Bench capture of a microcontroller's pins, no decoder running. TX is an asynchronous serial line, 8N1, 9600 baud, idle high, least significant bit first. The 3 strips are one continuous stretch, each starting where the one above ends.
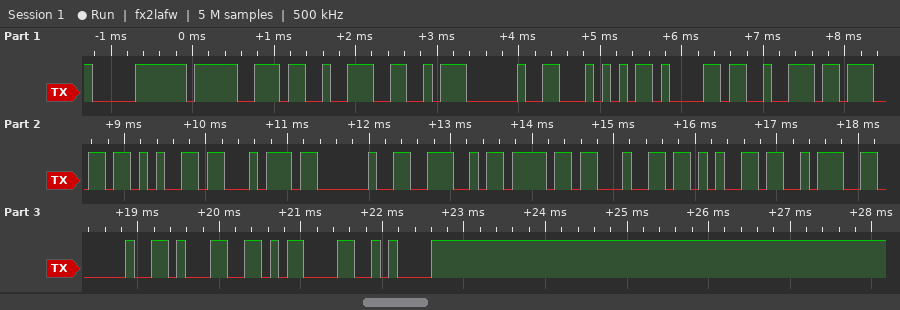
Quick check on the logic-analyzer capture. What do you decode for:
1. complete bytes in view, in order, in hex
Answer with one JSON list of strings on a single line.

["0xF0 0x9F 0x93 0xA6 0x20 0x54 0x61 0x72 0x67 0x65 0x74 0x20 0x4E 0x6F 0x64 0x65 0x3A 0x20 0x31 0x0D 0x0A"]
